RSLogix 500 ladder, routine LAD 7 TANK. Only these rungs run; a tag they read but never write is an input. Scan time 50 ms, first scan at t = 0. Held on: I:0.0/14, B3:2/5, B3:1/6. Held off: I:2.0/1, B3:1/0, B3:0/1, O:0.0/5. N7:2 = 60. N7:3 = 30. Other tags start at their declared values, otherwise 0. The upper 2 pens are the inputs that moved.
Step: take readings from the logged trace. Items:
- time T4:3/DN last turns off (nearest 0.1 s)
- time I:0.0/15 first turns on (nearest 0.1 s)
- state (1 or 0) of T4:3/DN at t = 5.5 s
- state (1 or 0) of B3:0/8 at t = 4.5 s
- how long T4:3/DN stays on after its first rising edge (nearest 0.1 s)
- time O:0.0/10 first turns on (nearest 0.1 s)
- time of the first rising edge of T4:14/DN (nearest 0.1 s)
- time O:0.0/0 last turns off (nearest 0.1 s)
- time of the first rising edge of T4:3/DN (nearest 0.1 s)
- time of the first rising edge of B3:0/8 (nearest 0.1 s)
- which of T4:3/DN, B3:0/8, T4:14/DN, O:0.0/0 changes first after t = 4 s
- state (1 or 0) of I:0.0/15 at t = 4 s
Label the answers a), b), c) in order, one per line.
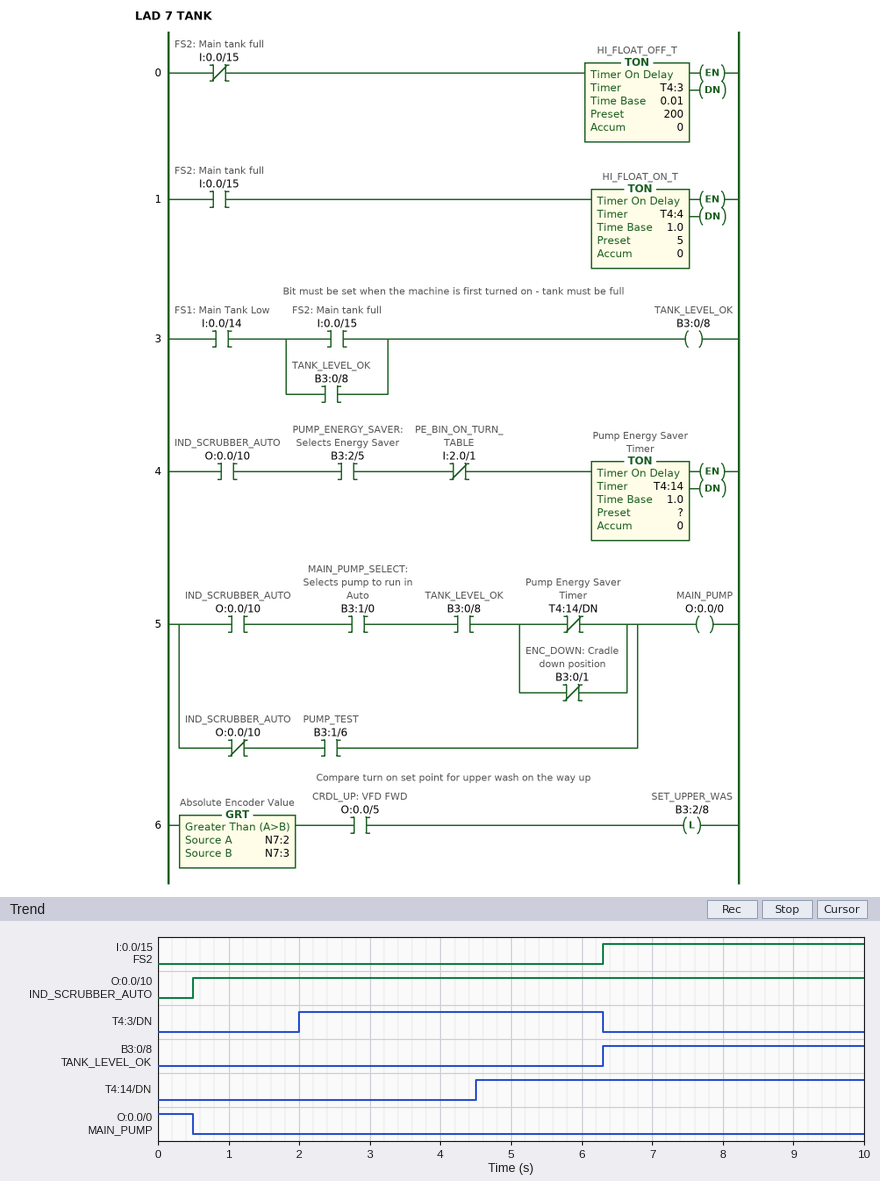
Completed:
a) 6.3 s
b) 6.3 s
c) 1
d) 0
e) 4.3 s
f) 0.5 s
g) 4.5 s
h) 0.5 s
i) 2.0 s
j) 6.3 s
k) T4:14/DN
l) 0
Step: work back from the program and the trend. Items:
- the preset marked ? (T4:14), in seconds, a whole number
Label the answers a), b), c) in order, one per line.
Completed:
a) 4 s
